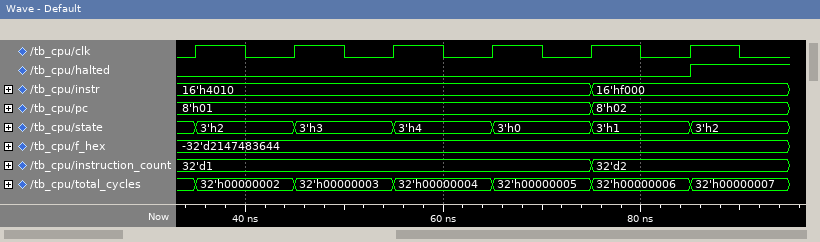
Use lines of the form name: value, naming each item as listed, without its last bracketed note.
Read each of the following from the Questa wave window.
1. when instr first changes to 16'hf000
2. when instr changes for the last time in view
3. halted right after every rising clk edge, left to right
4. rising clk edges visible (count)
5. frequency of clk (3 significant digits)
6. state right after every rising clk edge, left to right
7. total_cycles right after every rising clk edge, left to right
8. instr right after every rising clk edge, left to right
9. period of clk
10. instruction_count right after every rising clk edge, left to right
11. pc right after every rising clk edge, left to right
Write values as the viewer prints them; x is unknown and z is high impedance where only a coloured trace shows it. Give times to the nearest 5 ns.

when instr first changes to 16'hf000: 75 ns
when instr changes for the last time in view: 75 ns
halted right after every rising clk edge, left to right: 0 0 0 0 0 1
rising clk edges visible: 6
frequency of clk: 100 MHz
state right after every rising clk edge, left to right: 3'h2, 3'h3, 3'h4, 3'h0, 3'h1, 3'h2
total_cycles right after every rising clk edge, left to right: 32'h00000002, 32'h00000003, 32'h00000004, 32'h00000005, 32'h00000006, 32'h00000007
instr right after every rising clk edge, left to right: 16'h4010, 16'h4010, 16'h4010, 16'h4010, 16'hf000, 16'hf000
period of clk: 10 ns
instruction_count right after every rising clk edge, left to right: 32'd1, 32'd1, 32'd1, 32'd1, 32'd2, 32'd2
pc right after every rising clk edge, left to right: 8'h01, 8'h01, 8'h01, 8'h01, 8'h02, 8'h02
